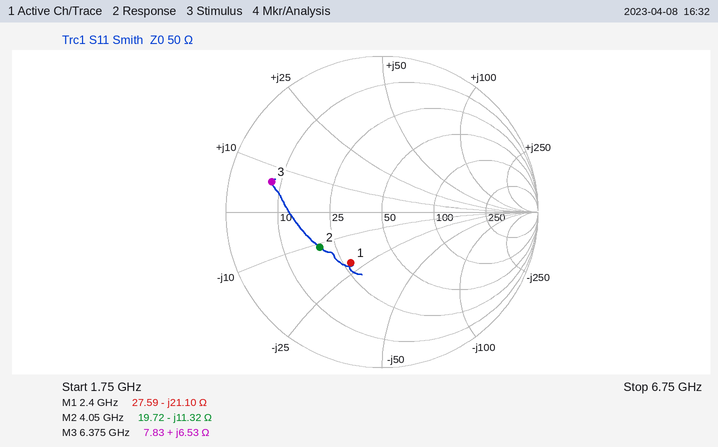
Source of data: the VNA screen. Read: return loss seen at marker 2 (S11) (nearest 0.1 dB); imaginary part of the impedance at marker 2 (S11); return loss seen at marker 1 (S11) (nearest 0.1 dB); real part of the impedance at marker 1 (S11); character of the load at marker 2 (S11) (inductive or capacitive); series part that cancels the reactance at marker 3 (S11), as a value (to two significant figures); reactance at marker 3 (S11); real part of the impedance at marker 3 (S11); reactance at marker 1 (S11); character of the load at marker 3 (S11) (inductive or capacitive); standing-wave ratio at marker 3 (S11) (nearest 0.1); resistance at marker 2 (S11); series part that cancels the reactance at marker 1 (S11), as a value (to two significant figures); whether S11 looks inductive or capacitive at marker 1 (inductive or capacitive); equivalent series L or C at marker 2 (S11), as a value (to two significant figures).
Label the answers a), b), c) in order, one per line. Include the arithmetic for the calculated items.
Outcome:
a) 6.8 dB
b) -11.32 Ω
c) 8.3 dB
d) 27.59 Ω
e) capacitive
f) C = 1/(2π × 6.375 GHz × 6.53 Ω) ≈ 3.8 pF
g) +6.53 Ω
h) 7.83 Ω
i) -21.10 Ω
j) inductive
k) 6.5
l) 19.72 Ω
m) L = 21.1 Ω/(2π × 2.4 GHz) ≈ 1.4 nH
n) capacitive
o) C = 1/(2π × 4.05 GHz × 11.32 Ω) ≈ 3.5 pF
